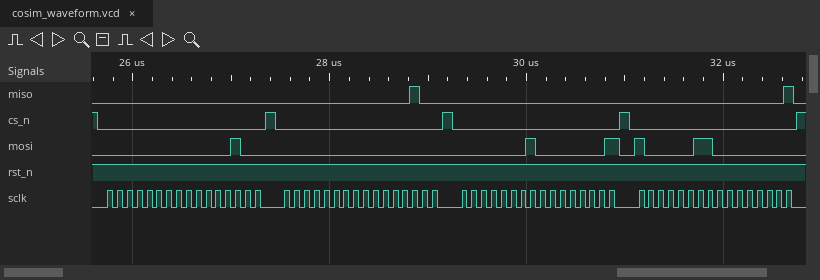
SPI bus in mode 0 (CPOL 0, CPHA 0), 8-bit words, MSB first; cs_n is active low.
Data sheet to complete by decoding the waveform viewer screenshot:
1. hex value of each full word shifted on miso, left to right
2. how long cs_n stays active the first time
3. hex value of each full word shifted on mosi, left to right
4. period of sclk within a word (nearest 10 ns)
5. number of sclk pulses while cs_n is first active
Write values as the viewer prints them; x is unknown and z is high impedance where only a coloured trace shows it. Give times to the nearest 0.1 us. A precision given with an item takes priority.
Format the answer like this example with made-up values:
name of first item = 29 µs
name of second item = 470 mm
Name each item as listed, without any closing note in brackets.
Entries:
hex value of each full word shifted on miso, left to right = 00, 00, 00, 04, 00, 00, 00, 01
how long cs_n stays active the first time = 1.7 us
hex value of each full word shifted on mosi, left to right = 00, 04, 00, 00, 01, 01, 83, 00
period of sclk within a word = 100 ns
number of sclk pulses while cs_n is first active = 16
